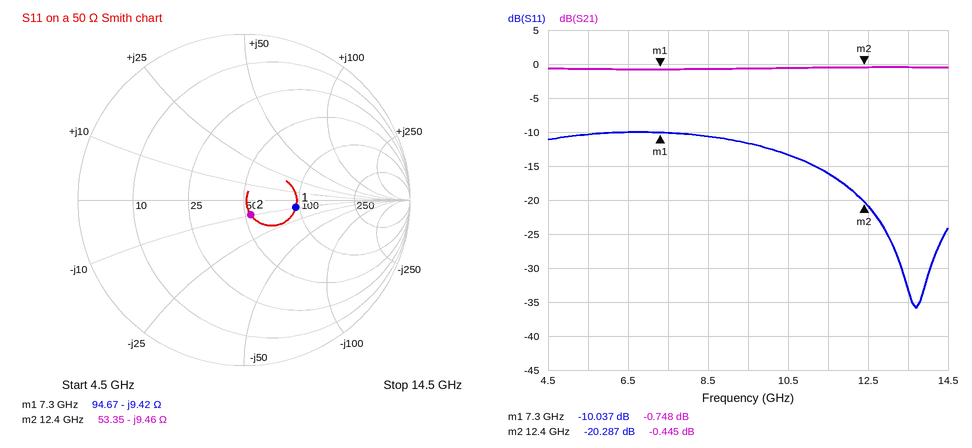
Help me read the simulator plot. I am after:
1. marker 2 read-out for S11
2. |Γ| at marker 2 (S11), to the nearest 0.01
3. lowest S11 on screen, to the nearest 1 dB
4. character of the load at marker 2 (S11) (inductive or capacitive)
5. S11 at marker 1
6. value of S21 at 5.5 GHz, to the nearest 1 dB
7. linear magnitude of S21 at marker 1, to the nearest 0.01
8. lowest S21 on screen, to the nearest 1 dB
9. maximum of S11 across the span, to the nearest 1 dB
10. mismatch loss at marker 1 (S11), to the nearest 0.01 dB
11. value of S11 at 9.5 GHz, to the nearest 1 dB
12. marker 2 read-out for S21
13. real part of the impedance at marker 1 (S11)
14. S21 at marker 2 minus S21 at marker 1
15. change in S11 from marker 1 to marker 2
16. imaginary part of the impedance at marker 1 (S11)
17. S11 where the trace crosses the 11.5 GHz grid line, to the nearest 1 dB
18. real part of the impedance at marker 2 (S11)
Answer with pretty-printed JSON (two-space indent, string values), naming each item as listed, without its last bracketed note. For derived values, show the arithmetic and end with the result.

{
  "marker 2 read-out for S11": "-20.287 dB",
  "|Γ| at marker 2 (S11), to the nearest 0.01": "0.10",
  "lowest S11 on screen, to the nearest 1 dB": "-36 dB",
  "character of the load at marker 2 (S11)": "capacitive",
  "S11 at marker 1": "-10.037 dB",
  "value of S21 at 5.5 GHz, to the nearest 1 dB": "-1 dB",
  "linear magnitude of S21 at marker 1, to the nearest 0.01": "10^(-0.748/20) ≈ 0.92",
  "lowest S21 on screen, to the nearest 1 dB": "-1 dB",
  "maximum of S11 across the span, to the nearest 1 dB": "-10 dB",
  "mismatch loss at marker 1 (S11), to the nearest 0.01 dB": "−10 log10(1 − 10^(-10.037/10)) ≈ 0.45 dB",
  "value of S11 at 9.5 GHz, to the nearest 1 dB": "-12 dB",
  "marker 2 read-out for S21": "-0.445 dB",
  "real part of the impedance at marker 1": "94.67 Ω",
  "S21 at marker 2 minus S21 at marker 1": "-0.445 − (-0.748) = 0.303 dB",
  "change in S11 from marker 1 to marker 2": "-20.287 − (-10.037) = -10.250 dB",
  "imaginary part of the impedance at marker 1": "-9.42 Ω",
  "S11 where the trace crosses the 11.5 GHz grid line, to the nearest 1 dB": "-16 dB",
  "real part of the impedance at marker 2": "53.35 Ω"
}
